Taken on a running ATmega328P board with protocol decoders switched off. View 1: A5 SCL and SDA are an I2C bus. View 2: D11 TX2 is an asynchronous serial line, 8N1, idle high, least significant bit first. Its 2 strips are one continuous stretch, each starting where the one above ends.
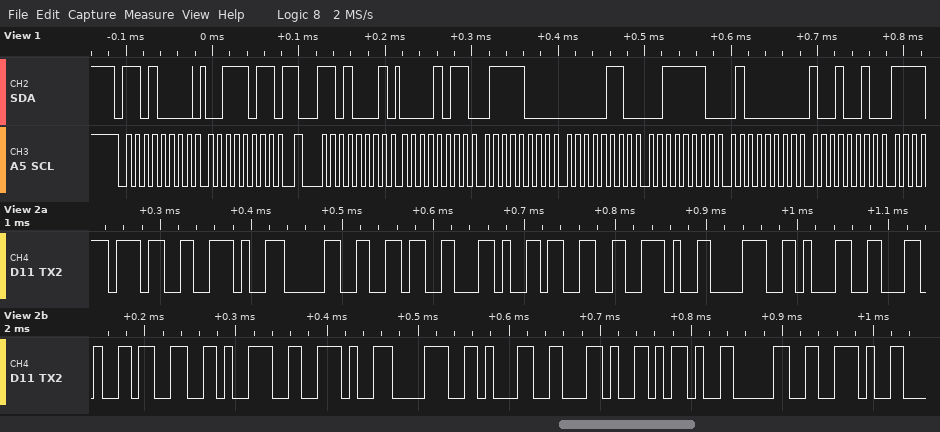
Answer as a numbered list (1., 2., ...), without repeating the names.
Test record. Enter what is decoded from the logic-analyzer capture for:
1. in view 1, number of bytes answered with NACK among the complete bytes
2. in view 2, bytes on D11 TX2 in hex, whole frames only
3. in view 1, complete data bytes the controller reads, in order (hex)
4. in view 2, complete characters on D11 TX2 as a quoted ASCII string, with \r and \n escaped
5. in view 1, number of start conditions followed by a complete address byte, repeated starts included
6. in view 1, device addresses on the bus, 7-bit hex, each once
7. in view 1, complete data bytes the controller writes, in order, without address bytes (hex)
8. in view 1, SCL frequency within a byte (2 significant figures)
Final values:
1. 0
2. 37 2E 30 36 2C 33 2E 38 31 2C 33 39 2E 38 31 2C 2D 30 2E
3. 0B 78 06 3E 40 92
4. "7.06,3.81,39.81,-0."
5. 2
6. 0x68
7. 3B
8. 100 kHz
